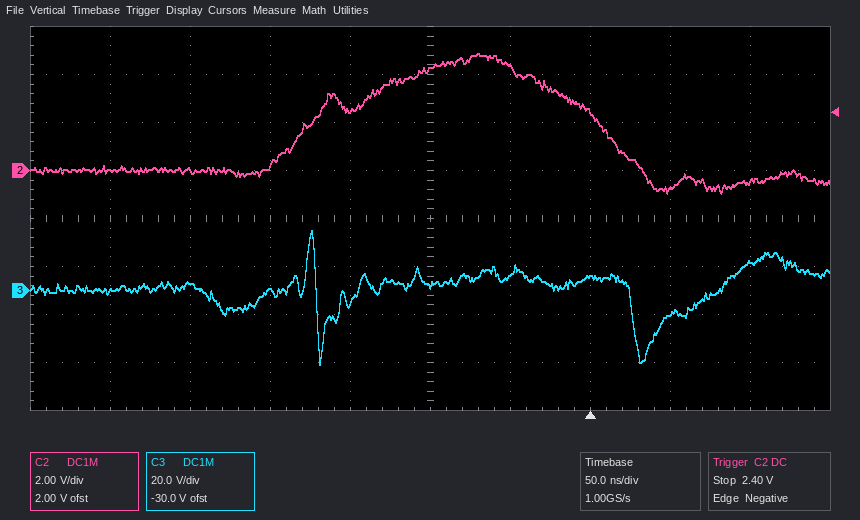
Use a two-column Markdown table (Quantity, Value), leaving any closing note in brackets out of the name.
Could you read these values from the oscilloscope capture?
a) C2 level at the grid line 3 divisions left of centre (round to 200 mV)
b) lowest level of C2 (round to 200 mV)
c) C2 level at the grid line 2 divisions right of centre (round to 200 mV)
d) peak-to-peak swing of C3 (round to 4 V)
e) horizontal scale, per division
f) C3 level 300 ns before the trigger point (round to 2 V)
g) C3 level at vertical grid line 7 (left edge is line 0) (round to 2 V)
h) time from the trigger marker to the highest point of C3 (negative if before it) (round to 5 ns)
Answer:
| Quantity | Value |
|---|---|
| C2 level at the grid line 3 divisions left of centre | 0.0 V |
| lowest level of C2 | -1.0 V |
| C2 level at the grid line 2 divisions right of centre | 2.4 V |
| peak-to-peak swing of C3 | 56 V |
| horizontal scale, per division | 50 ns |
| C3 level 300 ns before the trigger point | 0 V |
| C3 level at vertical grid line 7 (left edge is line 0) | 6 V |
| time from the trigger marker to the highest point of C3 (negative if before it) | -175 ns |
